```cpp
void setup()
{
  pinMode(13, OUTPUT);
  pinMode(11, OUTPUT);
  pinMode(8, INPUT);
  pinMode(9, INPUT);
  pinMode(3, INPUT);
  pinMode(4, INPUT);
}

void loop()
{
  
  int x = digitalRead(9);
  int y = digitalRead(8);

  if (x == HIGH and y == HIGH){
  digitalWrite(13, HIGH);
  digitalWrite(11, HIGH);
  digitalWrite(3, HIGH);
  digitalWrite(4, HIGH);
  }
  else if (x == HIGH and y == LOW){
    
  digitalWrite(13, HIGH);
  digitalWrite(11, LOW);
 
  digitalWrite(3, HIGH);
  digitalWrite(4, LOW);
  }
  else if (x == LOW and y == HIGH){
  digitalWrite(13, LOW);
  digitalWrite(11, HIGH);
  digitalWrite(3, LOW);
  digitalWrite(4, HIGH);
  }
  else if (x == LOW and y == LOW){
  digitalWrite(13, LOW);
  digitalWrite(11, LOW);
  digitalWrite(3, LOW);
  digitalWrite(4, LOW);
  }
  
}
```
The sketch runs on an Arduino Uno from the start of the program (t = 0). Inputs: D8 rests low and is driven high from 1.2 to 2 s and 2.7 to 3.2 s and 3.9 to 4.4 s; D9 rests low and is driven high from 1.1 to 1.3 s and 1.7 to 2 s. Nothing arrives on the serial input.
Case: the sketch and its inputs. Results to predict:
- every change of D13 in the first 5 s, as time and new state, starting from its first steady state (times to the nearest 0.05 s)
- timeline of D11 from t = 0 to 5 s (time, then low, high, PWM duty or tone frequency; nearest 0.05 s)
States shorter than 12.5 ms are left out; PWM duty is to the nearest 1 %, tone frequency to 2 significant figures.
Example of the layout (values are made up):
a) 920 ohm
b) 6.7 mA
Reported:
a) 0 s low; 1.1 s high; 1.3 s low; 1.7 s high; 2 s low
b) 0 s low; 1.2 s high; 2 s low; 2.7 s high; 3.2 s low; 3.9 s high; 4.4 s low
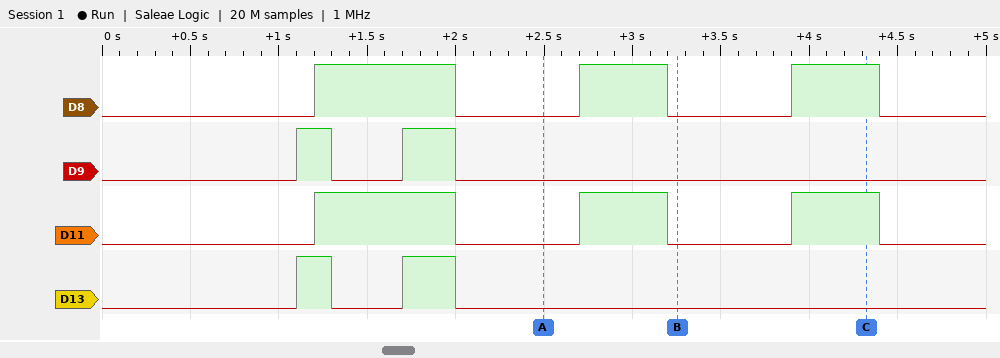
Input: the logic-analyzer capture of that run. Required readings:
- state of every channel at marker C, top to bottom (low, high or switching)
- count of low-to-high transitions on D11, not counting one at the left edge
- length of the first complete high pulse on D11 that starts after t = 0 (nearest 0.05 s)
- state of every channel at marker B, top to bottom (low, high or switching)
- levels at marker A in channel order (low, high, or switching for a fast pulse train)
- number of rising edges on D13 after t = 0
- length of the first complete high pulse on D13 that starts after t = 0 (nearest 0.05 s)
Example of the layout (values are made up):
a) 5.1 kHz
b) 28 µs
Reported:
a) D8 high, D9 low, D11 high, D13 low
b) 3
c) 0.80 s
d) D8 low, D9 low, D11 low, D13 low
e) D8 low, D9 low, D11 low, D13 low
f) 2
g) 0.20 s
